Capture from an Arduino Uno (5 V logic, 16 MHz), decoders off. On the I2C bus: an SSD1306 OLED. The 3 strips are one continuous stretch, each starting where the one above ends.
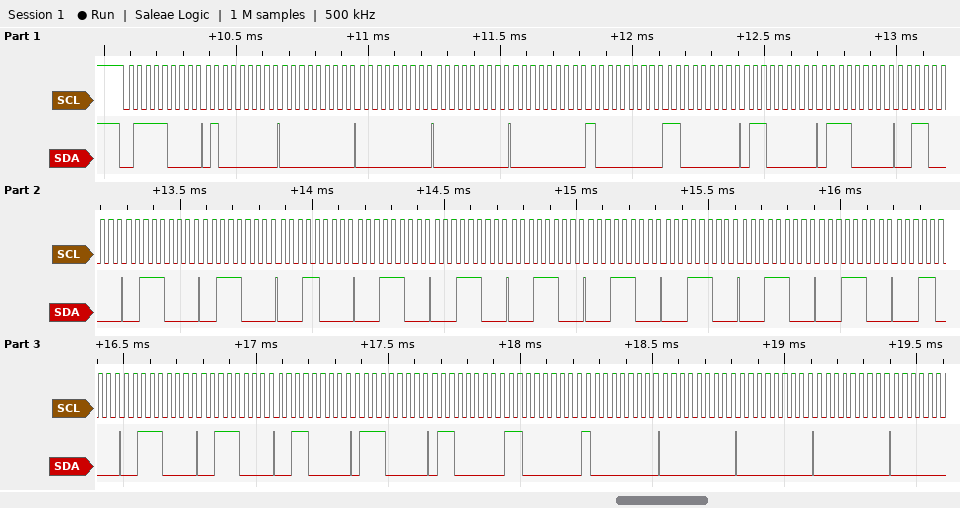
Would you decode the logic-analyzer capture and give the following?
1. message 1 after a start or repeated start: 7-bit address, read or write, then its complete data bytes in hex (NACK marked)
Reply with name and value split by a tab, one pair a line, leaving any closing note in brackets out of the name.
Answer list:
message 1 after a start or repeated start: 7-bit address, read or write, then its complete data bytes in hex	0x3C write: 40 00 00 00 00 80 C0 60 70 30 38 38 18 1C 1C 1C 1C 1C 1C 1C 18 38 38 30 70 60 C0 80 00 00 00
